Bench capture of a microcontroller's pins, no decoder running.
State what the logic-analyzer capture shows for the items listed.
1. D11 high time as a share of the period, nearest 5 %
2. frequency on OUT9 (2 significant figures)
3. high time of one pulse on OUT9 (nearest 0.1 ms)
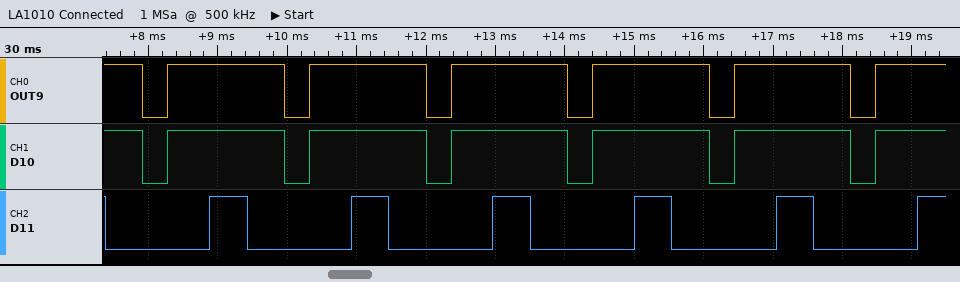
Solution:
25 %
490 Hz
1.7 ms
